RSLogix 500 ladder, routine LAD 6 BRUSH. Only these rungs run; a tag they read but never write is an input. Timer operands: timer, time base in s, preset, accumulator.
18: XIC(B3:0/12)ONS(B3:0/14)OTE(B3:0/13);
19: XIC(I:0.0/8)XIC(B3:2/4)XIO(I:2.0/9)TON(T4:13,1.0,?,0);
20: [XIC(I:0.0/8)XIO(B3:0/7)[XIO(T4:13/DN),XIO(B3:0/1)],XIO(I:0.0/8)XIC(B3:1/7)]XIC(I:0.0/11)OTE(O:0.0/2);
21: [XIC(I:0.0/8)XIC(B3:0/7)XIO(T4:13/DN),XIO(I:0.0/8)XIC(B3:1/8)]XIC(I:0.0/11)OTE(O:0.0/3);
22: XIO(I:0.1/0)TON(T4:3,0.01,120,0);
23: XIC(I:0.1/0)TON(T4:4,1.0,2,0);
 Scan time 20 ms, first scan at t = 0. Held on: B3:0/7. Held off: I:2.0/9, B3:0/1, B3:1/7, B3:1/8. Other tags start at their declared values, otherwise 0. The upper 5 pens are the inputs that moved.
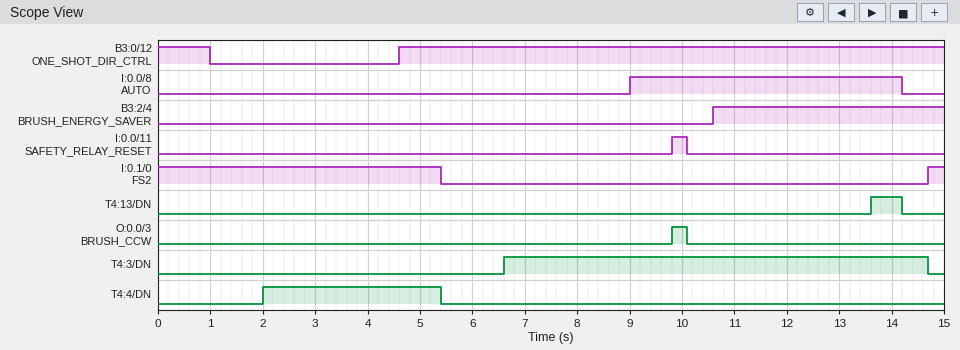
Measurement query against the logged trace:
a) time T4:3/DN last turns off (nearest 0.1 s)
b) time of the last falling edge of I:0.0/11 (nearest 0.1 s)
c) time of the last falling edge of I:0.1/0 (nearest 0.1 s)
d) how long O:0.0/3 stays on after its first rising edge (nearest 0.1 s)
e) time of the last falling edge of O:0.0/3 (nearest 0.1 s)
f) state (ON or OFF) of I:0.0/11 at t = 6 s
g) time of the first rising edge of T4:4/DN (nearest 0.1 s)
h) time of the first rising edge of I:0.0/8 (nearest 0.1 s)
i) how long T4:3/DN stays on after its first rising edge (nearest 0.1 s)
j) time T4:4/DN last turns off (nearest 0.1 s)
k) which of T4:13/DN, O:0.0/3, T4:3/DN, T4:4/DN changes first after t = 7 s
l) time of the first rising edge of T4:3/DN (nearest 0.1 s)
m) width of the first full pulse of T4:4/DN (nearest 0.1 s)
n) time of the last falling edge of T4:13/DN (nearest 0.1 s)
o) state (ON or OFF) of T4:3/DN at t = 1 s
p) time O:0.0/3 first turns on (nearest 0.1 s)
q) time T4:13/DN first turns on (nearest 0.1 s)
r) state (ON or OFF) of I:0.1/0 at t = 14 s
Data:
14.7 s
10.1 s
5.4 s
0.3 s
10.1 s
OFF
2.0 s
9.0 s
8.1 s
5.4 s
O:0.0/3
6.6 s
3.4 s
14.2 s
OFF
9.8 s
13.6 s
OFF
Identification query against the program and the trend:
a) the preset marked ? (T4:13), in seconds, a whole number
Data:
3 s
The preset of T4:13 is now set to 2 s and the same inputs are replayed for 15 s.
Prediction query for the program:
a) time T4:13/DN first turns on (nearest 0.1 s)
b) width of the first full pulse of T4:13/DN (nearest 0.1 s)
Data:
12.6 s
1.6 s
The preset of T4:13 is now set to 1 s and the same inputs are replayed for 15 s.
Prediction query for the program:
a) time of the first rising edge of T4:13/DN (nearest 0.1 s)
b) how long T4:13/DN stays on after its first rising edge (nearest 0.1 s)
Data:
11.6 s
2.6 s
